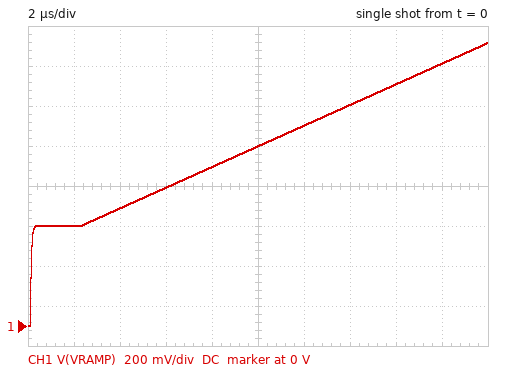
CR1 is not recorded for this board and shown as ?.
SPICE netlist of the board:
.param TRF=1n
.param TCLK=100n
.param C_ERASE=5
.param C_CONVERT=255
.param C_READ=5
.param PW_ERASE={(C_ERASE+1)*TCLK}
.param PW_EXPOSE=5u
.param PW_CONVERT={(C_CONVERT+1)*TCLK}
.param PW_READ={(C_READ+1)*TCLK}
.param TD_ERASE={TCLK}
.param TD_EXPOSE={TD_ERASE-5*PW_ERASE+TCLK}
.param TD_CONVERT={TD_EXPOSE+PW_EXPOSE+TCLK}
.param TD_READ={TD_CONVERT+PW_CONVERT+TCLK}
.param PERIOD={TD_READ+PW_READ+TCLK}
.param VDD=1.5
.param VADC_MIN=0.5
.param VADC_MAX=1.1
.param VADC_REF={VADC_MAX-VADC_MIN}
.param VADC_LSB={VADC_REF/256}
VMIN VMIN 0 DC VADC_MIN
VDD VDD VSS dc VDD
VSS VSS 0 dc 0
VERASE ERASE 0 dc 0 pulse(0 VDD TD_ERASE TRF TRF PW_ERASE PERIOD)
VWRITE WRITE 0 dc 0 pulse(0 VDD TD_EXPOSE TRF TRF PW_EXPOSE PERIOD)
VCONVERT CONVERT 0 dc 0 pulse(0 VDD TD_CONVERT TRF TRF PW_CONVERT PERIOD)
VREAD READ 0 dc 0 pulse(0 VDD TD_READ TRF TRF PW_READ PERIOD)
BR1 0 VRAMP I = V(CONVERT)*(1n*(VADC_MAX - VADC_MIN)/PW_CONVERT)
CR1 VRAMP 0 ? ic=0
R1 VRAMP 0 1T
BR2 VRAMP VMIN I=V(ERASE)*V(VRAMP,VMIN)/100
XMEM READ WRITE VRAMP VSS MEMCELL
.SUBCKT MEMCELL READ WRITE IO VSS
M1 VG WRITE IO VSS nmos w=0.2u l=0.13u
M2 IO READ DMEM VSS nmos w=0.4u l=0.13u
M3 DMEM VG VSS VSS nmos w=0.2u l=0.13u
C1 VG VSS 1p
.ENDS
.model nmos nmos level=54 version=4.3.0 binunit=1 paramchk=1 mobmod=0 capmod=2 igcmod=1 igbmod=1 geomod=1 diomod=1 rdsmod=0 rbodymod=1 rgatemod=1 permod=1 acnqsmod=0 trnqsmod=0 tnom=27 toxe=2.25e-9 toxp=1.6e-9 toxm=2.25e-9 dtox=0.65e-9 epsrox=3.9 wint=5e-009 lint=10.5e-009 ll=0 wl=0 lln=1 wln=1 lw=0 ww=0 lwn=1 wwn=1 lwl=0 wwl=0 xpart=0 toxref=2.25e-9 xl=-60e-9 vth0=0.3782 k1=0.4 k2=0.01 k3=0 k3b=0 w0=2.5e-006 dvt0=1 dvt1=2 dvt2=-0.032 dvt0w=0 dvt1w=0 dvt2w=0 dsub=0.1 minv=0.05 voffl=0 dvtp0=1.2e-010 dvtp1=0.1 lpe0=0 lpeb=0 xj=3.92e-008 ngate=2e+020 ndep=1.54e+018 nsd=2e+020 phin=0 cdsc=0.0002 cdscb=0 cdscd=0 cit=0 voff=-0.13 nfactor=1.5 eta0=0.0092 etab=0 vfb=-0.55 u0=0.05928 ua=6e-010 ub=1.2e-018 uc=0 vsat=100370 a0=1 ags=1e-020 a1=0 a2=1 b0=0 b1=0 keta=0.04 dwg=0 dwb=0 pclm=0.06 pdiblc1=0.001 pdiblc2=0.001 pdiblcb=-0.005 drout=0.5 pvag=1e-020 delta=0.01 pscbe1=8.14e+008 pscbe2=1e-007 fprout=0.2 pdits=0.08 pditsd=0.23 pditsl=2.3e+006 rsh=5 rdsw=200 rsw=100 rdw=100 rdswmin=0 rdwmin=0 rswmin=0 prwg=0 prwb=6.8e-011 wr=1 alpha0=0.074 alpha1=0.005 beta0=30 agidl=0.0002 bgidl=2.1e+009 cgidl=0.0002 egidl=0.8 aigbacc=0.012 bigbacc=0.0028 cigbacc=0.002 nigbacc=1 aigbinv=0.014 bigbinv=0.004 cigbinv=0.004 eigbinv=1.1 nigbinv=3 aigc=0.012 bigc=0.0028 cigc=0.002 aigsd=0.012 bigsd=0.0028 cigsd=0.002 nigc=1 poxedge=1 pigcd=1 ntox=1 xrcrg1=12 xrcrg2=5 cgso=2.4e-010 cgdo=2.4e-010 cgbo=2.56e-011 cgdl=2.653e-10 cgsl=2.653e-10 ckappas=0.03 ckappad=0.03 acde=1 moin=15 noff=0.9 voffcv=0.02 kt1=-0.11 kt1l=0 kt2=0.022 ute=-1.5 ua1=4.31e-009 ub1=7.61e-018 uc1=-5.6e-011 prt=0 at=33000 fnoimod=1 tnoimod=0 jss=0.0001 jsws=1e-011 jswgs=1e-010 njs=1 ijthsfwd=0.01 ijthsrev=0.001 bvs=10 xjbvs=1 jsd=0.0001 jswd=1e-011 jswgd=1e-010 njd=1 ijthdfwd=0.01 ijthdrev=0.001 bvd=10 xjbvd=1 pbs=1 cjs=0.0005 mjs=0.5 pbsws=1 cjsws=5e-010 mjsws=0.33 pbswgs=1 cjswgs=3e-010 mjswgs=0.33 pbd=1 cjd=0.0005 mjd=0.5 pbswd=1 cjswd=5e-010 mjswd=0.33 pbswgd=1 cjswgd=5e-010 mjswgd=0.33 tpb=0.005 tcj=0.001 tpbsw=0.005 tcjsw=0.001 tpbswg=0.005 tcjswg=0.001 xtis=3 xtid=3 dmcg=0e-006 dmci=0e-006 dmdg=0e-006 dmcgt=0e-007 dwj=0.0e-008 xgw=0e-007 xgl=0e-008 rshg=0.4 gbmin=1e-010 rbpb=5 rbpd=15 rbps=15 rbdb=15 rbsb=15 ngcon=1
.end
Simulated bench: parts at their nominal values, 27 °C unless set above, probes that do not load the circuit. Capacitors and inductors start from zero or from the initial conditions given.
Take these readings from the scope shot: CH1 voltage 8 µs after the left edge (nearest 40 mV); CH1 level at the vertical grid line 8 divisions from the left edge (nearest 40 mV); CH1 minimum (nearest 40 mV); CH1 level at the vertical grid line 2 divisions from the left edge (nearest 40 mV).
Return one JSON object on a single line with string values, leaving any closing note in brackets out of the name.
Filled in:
{"CH1 voltage 8 µs after the left edge": "800 mV", "CH1 level at the vertical grid line 8 divisions from the left edge": "1.20 V", "CH1 minimum": "0 V", "CH1 level at the vertical grid line 2 divisions from the left edge": "600 mV"}
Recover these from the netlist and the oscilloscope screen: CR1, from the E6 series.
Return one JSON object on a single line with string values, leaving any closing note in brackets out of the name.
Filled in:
{"CR1, from the E6 series": "680 pF"}
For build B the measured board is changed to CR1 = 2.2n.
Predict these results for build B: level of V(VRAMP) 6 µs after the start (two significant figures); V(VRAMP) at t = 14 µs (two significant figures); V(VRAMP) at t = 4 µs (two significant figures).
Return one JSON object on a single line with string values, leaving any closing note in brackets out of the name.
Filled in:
{"level of V(VRAMP) 6 µs after the start": "550 mV", "V(VRAMP) at t = 14 µs": "680 mV", "V(VRAMP) at t = 4 µs": "520 mV"}
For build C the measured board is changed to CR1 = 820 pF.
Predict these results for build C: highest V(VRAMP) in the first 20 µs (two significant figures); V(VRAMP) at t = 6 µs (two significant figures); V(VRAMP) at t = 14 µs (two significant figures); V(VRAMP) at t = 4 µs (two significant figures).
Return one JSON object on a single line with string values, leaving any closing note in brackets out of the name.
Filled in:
{"highest V(VRAMP) in the first 20 µs": "1.3 V", "V(VRAMP) at t = 6 µs": "660 mV", "V(VRAMP) at t = 14 µs": "1.0 V", "V(VRAMP) at t = 4 µs": "570 mV"}
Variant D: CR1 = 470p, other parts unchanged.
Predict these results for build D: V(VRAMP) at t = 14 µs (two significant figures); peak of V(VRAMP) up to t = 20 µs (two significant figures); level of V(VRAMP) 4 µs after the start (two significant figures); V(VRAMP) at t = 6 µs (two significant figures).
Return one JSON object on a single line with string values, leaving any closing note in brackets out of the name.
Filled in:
{"V(VRAMP) at t = 14 µs": "1.4 V", "peak of V(VRAMP) up to t = 20 µs": "1.8 V", "level of V(VRAMP) 4 µs after the start": "630 mV", "V(VRAMP) at t = 6 µs": "780 mV"}
